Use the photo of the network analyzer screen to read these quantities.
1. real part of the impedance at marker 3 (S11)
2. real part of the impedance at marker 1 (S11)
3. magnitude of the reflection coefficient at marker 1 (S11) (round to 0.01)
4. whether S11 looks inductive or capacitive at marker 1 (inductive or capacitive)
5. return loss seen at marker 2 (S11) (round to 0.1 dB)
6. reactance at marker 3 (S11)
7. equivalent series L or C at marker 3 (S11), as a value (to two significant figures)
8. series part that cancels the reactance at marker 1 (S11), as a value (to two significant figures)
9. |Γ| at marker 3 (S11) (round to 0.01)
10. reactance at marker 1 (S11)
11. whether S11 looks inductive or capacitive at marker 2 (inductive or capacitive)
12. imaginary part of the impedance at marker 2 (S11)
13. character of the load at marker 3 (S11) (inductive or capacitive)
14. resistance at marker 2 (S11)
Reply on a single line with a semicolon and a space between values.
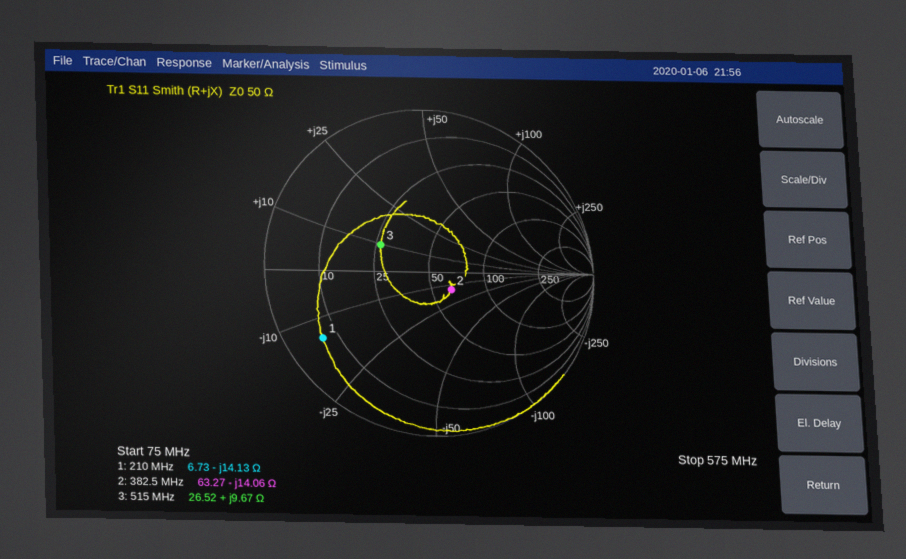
26.52 Ω; 6.73 Ω; 0.78; capacitive; 15.4 dB; +9.67 Ω; 3.0 nH; 11 nH; 0.33; -14.13 Ω; capacitive; -14.06 Ω; inductive; 63.27 Ω
